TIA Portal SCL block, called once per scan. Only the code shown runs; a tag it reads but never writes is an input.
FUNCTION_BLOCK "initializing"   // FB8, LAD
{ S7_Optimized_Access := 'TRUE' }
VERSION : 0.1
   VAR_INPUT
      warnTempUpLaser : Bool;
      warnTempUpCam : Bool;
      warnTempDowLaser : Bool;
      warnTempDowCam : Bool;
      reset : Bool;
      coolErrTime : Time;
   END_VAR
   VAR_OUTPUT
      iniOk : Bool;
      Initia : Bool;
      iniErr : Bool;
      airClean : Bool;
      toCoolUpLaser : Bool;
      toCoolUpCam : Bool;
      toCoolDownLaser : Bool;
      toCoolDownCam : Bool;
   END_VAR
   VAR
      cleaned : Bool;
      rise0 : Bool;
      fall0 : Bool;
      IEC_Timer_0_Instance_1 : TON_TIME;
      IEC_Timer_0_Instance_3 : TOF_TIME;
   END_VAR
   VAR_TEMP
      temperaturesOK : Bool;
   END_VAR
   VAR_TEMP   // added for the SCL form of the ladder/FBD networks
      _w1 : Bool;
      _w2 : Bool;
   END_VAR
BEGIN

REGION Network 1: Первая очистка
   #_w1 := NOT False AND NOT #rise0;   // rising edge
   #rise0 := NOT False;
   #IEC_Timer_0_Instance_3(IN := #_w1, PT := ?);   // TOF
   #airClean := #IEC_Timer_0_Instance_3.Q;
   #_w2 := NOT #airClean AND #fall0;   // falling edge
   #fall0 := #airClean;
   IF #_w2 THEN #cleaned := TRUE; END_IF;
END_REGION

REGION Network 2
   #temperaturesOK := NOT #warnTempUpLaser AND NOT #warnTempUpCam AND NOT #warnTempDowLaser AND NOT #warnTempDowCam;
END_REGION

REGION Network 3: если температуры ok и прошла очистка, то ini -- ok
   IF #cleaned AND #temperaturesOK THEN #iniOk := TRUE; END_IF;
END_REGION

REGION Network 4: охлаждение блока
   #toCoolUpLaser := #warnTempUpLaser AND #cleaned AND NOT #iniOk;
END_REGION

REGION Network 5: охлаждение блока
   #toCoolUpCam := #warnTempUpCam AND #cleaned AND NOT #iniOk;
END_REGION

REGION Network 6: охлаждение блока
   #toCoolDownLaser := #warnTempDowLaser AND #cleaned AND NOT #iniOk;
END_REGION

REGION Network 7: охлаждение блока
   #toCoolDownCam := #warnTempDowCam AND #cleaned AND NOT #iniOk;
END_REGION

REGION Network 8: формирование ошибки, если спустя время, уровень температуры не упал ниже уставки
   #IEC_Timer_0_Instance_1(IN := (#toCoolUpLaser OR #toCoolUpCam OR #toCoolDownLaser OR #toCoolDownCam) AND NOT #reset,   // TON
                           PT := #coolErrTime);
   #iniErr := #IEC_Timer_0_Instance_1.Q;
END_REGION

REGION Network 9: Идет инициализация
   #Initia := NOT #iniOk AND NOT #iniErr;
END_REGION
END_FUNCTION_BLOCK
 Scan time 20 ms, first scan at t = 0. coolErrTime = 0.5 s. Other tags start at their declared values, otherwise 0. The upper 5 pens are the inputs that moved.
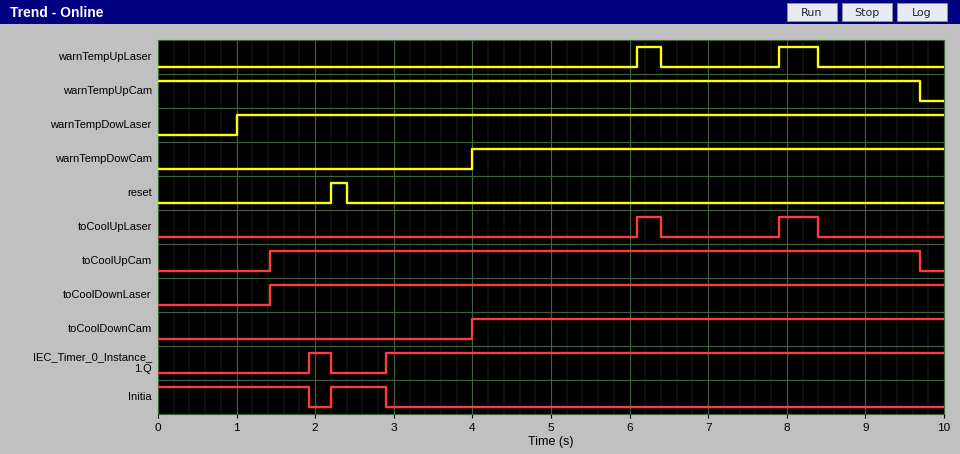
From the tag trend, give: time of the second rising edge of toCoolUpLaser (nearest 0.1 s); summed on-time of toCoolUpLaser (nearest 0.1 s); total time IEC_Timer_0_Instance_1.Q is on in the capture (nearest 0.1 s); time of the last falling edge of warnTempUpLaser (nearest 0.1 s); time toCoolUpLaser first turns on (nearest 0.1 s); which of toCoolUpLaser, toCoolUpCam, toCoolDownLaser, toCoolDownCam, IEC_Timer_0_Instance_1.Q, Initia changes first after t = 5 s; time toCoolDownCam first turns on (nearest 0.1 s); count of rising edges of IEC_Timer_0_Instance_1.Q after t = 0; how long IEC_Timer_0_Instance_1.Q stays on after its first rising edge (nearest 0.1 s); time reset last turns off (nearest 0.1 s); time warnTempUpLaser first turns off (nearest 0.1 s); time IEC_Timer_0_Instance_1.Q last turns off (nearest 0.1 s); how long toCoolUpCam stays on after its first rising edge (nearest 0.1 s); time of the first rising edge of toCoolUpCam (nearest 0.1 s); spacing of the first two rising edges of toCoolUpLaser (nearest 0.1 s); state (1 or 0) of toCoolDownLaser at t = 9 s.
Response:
7.9 s
0.8 s
7.4 s
8.4 s
6.1 s
toCoolUpLaser
4.0 s
2
0.3 s
2.4 s
6.4 s
2.2 s
8.3 s
1.4 s
1.8 s
1
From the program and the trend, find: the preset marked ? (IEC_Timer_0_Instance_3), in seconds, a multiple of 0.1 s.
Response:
1.4 s
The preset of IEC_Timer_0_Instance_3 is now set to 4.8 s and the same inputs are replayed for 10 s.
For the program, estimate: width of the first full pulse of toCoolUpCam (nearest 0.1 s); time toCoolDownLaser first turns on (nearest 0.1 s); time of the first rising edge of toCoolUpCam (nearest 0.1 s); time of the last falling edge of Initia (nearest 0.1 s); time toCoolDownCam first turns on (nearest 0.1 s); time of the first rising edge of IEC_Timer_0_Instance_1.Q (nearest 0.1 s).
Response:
4.9 s
4.8 s
4.8 s
5.3 s
4.8 s
5.3 s
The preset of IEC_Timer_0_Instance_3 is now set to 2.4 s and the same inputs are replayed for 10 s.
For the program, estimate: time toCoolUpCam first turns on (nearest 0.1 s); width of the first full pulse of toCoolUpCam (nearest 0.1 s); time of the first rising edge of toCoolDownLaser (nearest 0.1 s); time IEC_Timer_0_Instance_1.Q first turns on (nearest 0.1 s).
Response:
2.4 s
7.3 s
2.4 s
2.9 s
